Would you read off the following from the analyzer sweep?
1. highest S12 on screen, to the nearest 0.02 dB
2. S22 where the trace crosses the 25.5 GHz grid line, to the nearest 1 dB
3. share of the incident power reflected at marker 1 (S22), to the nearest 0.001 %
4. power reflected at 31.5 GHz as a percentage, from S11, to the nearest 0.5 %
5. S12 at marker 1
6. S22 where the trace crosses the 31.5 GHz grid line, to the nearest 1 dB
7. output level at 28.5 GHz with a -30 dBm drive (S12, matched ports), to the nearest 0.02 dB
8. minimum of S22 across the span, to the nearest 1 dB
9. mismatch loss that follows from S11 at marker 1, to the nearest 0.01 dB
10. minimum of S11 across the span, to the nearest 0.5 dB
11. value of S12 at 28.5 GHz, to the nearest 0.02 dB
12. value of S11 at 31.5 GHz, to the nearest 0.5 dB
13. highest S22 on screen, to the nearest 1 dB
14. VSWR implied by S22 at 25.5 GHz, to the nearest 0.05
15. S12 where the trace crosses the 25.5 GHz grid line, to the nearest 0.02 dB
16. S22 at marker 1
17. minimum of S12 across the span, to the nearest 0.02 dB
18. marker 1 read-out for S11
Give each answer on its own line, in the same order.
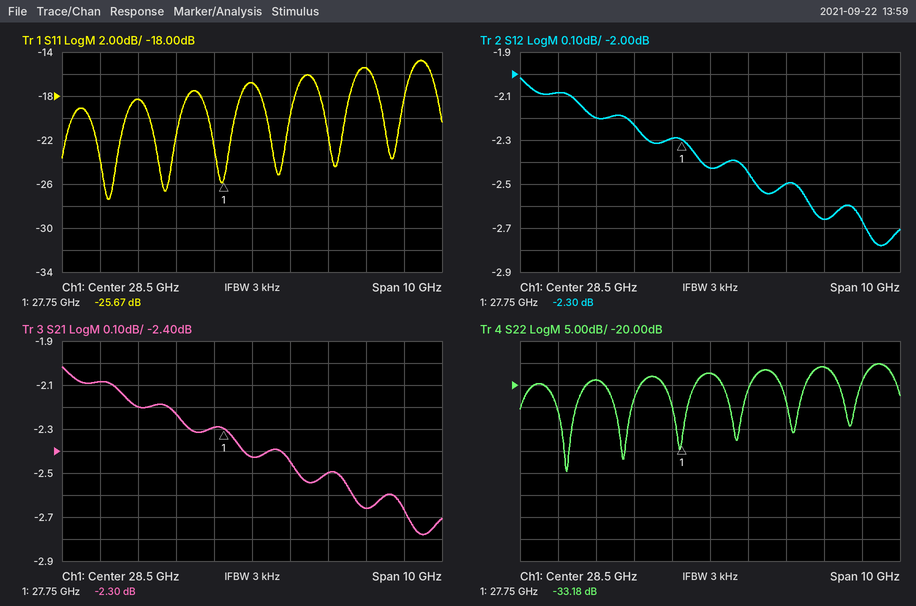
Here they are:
-2.02 dB
-19 dB
0.048 %
3.0 %
-2.30 dB
-16 dB
-32.42 dBm
-40 dB
0.01 dB
-27.5 dB
-2.42 dB
-15.5 dB
-15 dB
1.25
-2.20 dB
-33.18 dB
-2.78 dB
-25.67 dB
